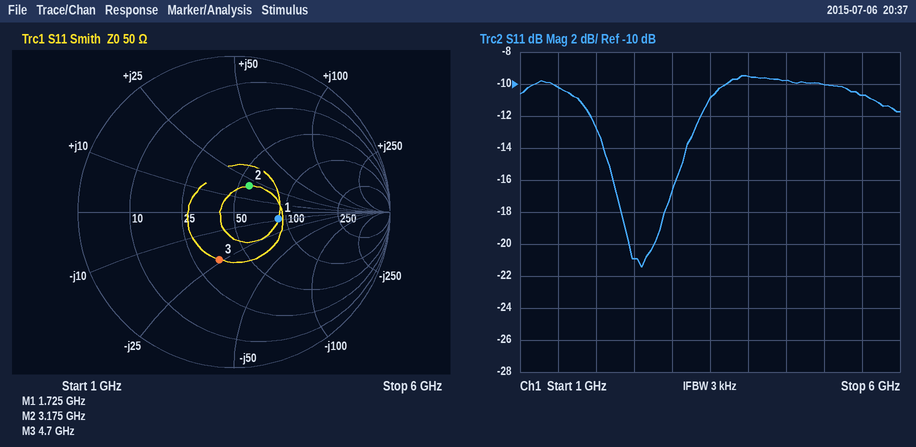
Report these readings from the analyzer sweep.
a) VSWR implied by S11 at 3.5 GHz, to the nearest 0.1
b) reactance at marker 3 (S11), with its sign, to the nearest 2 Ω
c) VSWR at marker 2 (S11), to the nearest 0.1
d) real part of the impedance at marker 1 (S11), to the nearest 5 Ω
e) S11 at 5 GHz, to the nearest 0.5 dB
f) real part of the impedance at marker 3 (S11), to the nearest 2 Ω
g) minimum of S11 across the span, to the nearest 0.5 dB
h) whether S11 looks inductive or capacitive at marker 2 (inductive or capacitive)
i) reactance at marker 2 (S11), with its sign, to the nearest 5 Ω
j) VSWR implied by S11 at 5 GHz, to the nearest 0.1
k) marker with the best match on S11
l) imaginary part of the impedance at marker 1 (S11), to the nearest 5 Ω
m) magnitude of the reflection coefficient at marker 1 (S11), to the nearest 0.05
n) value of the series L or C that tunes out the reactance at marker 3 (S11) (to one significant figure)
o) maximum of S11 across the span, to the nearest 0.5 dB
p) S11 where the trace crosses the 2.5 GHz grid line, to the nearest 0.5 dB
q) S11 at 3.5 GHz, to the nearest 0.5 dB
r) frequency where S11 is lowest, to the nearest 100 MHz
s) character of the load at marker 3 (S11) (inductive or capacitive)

1.8
-24 Ω
1.5
90 Ω
-10.0 dB
34 Ω
-21.5 dB
inductive
+20 Ω
1.9
marker 2
-10 Ω
0.30
800 pH
-9.5 dB
-21.0 dB
-11.0 dB
2.6 GHz
capacitive
